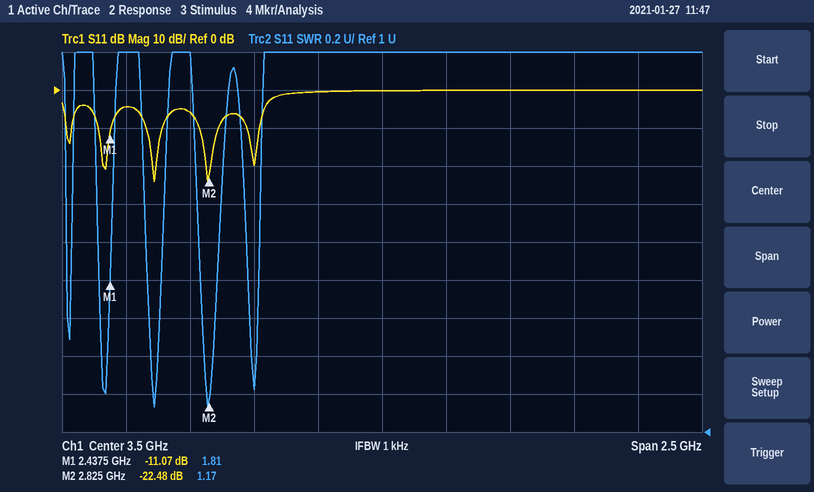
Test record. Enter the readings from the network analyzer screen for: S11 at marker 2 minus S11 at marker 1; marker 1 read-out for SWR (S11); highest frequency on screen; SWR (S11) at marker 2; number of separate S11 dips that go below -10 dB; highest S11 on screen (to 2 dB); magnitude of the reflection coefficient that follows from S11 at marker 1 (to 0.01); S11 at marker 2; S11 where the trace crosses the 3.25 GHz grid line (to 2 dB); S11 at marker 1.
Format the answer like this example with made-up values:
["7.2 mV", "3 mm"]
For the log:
["-11.41 dB", "1.81", "4.75 GHz", "1.17", "5", "0 dB", "0.28", "-22.48 dB", "0 dB", "-11.07 dB"]
